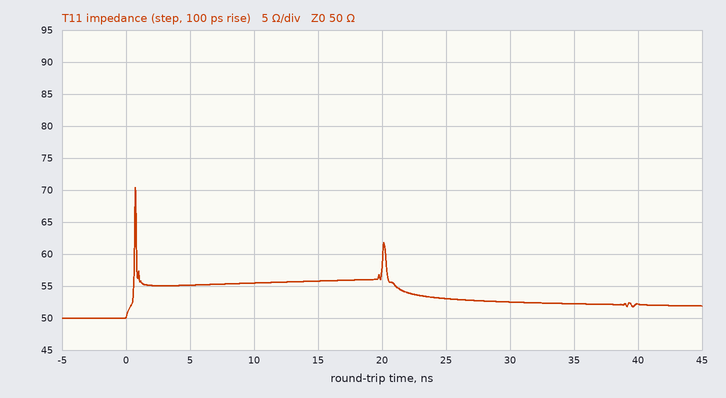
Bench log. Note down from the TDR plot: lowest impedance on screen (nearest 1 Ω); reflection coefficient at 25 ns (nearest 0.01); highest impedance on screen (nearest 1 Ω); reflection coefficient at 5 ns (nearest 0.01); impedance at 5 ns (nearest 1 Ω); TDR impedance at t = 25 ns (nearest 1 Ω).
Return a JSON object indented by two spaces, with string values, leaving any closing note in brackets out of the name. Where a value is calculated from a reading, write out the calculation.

{
  "lowest impedance on screen": "50 Ω",
  "reflection coefficient at 25 ns": "(53 − 50)/(53 + 50) ≈ +0.03",
  "highest impedance on screen": "70 Ω",
  "reflection coefficient at 5 ns": "(55 − 50)/(55 + 50) ≈ +0.05",
  "impedance at 5 ns": "55 Ω",
  "TDR impedance at t = 25 ns": "53 Ω"
}
